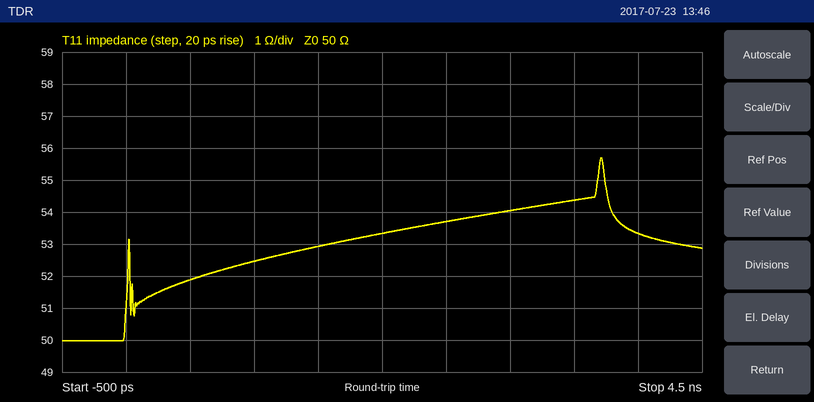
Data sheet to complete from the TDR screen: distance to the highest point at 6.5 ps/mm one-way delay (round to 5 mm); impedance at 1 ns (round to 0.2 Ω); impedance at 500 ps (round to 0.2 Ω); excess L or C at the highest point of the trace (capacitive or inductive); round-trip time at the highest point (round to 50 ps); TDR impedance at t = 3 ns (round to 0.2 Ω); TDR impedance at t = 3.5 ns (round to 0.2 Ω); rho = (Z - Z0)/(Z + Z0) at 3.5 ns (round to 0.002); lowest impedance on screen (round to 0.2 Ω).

285 mm
52.4 Ω
51.8 Ω
inductive
3.70 ns
54.0 Ω
54.4 Ω
+0.042
50.0 Ω
